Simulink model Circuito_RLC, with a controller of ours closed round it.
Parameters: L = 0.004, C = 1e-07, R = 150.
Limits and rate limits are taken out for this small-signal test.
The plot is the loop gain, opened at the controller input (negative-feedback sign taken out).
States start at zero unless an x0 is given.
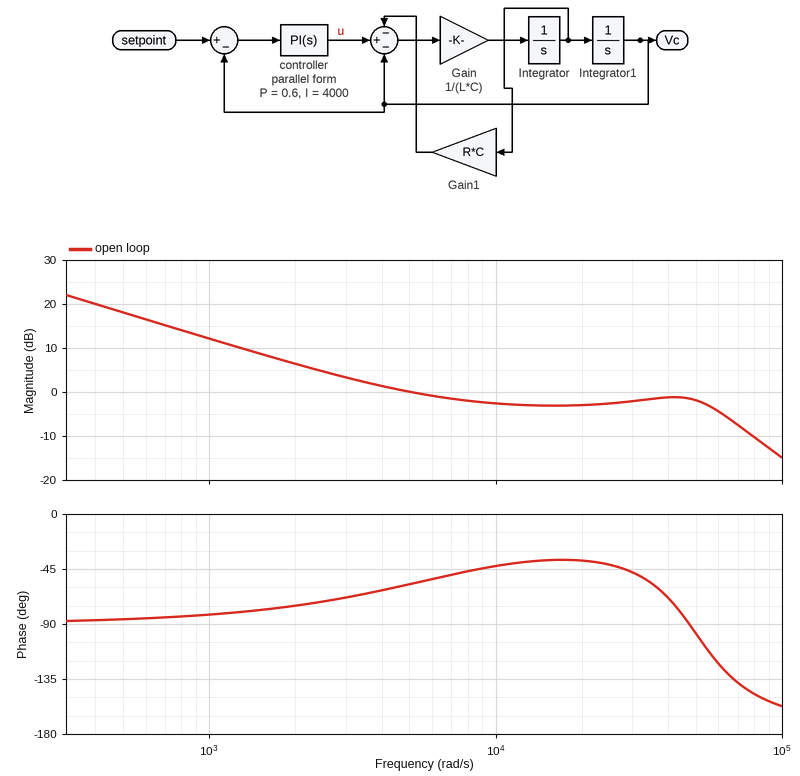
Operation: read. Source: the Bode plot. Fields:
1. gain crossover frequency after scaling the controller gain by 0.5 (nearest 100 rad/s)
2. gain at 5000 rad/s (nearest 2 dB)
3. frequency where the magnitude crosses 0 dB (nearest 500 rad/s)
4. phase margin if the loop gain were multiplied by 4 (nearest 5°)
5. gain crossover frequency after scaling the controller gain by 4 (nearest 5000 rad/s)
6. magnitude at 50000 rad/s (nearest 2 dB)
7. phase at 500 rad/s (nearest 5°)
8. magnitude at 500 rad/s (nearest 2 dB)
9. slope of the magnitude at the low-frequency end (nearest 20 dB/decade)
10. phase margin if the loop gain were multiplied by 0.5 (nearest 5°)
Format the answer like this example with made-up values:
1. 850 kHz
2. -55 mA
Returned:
1. 2100 rad/s
2. 0 dB
3. 5000 rad/s
4. 30°
5. 85000 rad/s
6. -2 dB
7. -85°
8. 18 dB
9. -20 dB/decade
10. 105°
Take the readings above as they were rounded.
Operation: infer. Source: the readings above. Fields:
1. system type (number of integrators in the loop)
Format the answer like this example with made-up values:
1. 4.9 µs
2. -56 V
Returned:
1. 1
